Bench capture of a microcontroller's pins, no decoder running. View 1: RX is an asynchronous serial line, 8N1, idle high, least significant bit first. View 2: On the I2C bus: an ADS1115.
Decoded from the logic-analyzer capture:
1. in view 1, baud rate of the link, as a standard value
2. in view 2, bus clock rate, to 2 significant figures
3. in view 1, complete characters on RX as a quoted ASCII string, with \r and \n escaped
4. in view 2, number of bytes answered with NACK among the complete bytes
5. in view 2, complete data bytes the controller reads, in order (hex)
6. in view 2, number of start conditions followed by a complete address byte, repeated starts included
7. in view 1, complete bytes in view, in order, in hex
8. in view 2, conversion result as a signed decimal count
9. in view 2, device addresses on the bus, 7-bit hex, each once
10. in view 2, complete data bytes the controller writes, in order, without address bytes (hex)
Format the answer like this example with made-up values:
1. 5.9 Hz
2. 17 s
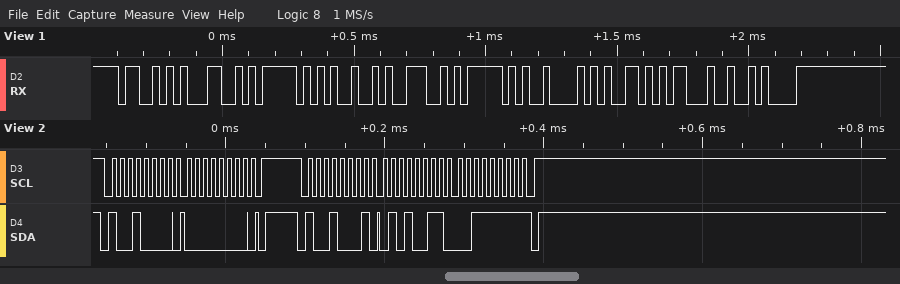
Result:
1. 38400 baud
2. 100 kHz
3. "SL_IN_BY#\n"
4. 1
5. 53 3F
6. 2
7. 53 4C 5F 49 4E 5F 42 59 23 0A
8. 21311
9. 0x48
10. 00
